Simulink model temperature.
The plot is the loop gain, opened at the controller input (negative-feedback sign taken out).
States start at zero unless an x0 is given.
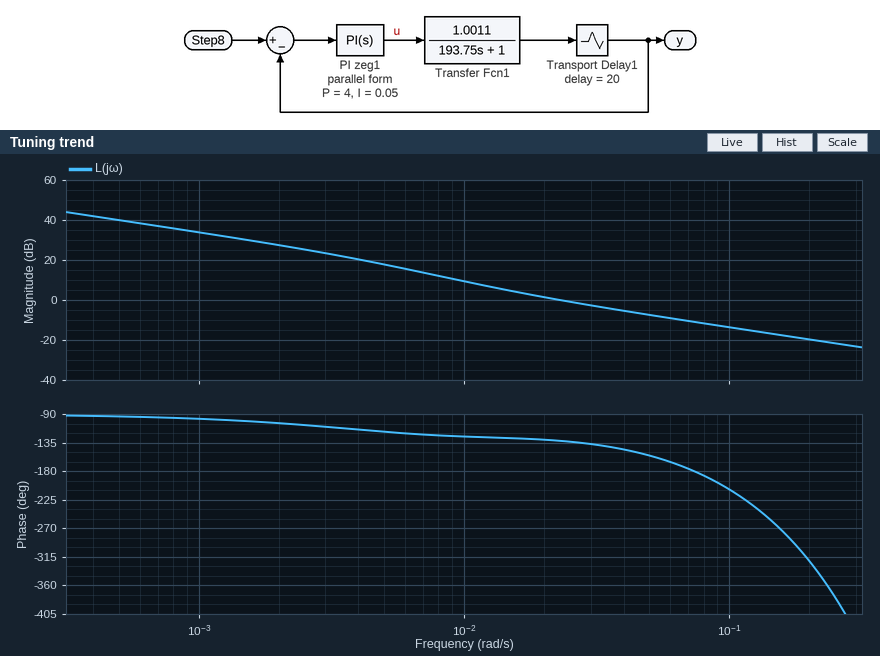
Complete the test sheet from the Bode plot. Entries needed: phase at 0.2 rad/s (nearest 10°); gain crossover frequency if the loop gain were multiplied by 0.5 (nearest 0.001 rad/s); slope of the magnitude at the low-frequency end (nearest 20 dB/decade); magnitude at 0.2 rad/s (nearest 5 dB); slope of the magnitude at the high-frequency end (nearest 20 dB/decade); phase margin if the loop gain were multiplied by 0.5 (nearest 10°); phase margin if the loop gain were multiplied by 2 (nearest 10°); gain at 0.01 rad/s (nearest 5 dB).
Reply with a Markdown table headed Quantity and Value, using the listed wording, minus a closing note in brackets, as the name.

| Quantity | Value |
|---|---|
| phase at 0.2 rad/s | -320° |
| gain crossover frequency if the loop gain were multiplied by 0.5 | 0.013 rad/s |
| slope of the magnitude at the low-frequency end | -20 dB/decade |
| magnitude at 0.2 rad/s | -20 dB |
| slope of the magnitude at the high-frequency end | -20 dB/decade |
| phase margin if the loop gain were multiplied by 0.5 | 50° |
| phase margin if the loop gain were multiplied by 2 | 30° |
| gain at 0.01 rad/s | 10 dB |
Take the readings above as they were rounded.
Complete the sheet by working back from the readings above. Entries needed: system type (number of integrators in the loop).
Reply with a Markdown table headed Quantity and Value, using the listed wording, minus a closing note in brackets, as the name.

| Quantity | Value |
|---|---|
| system type | 1 |
